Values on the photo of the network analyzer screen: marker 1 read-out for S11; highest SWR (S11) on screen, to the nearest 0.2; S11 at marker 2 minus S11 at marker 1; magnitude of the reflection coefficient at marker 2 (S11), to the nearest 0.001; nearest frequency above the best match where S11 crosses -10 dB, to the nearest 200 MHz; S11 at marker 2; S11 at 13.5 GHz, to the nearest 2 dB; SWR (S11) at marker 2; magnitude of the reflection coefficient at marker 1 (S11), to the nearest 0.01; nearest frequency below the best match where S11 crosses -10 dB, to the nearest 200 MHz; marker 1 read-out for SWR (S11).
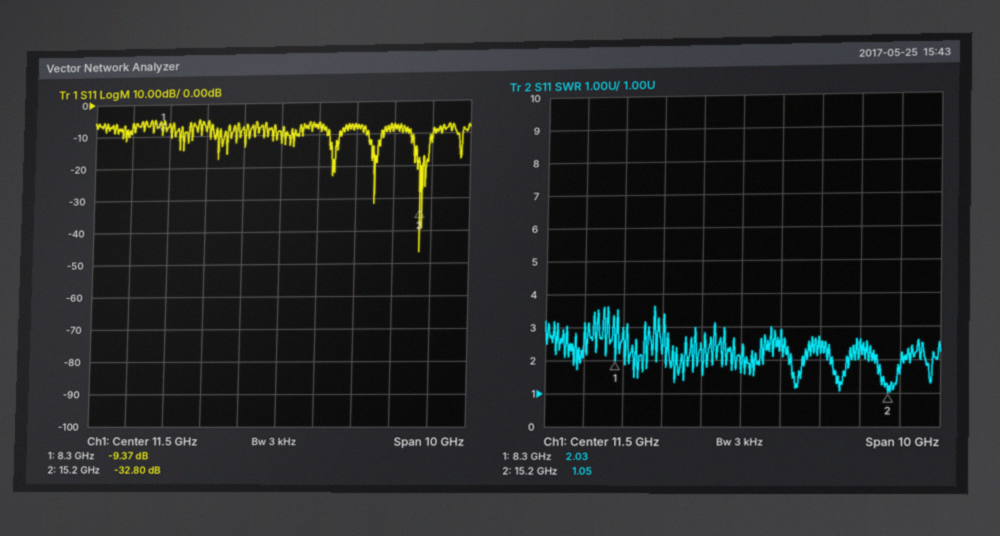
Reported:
-9.37 dB
3.6
-23.43 dB
0.023
15.6 GHz
-32.80 dB
-8 dB
1.05
0.34
15.0 GHz
2.03
